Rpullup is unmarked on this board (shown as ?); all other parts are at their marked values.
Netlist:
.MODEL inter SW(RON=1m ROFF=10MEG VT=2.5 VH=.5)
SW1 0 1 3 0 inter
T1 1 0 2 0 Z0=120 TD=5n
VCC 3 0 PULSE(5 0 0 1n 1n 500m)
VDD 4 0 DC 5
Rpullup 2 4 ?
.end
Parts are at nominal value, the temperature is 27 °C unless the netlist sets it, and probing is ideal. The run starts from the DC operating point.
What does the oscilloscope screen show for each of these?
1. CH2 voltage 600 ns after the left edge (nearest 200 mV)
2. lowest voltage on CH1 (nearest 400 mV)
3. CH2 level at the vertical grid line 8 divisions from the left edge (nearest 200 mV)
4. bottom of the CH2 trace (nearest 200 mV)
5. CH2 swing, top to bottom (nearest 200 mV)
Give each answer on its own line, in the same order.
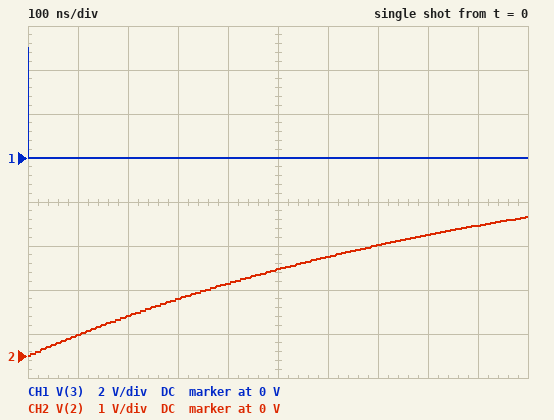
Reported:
2.2 V
0 V
2.8 V
0 V
3.2 V
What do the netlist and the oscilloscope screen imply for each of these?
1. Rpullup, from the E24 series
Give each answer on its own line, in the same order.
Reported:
24 kΩ
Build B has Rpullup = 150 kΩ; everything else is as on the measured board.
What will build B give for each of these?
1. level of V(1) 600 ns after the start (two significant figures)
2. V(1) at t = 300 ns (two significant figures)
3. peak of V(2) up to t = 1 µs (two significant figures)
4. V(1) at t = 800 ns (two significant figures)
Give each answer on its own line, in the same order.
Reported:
450 mV
230 mV
740 mV
600 mV
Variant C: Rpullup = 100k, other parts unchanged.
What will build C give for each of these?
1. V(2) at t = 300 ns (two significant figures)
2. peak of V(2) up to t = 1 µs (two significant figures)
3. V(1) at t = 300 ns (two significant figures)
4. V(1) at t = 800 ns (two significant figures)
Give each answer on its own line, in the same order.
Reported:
350 mV
1.1 V
340 mV
870 mV
